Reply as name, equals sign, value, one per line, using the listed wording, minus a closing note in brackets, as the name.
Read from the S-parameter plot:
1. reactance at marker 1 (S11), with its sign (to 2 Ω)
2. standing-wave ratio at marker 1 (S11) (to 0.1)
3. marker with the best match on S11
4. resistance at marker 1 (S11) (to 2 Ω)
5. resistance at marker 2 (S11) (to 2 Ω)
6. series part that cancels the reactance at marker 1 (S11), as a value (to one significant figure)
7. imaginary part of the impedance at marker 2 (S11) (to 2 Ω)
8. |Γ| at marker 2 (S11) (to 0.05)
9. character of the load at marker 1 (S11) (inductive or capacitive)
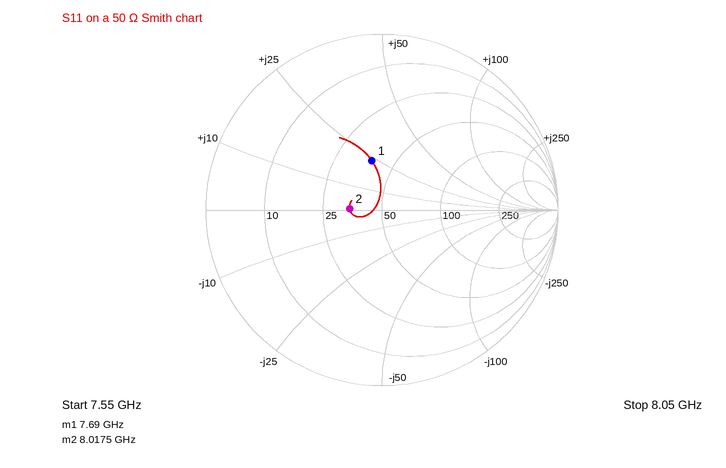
reactance at marker 1 (S11), with its sign = +24 Ω
standing-wave ratio at marker 1 (S11) = 1.8
marker with the best match on S11 = marker 2
resistance at marker 1 (S11) = 38 Ω
resistance at marker 2 (S11) = 34 Ω
series part that cancels the reactance at marker 1 (S11), as a value = 900 fF
imaginary part of the impedance at marker 2 (S11) = 0 Ω
|Γ| at marker 2 (S11) = 0.20
character of the load at marker 1 (S11) = inductive
